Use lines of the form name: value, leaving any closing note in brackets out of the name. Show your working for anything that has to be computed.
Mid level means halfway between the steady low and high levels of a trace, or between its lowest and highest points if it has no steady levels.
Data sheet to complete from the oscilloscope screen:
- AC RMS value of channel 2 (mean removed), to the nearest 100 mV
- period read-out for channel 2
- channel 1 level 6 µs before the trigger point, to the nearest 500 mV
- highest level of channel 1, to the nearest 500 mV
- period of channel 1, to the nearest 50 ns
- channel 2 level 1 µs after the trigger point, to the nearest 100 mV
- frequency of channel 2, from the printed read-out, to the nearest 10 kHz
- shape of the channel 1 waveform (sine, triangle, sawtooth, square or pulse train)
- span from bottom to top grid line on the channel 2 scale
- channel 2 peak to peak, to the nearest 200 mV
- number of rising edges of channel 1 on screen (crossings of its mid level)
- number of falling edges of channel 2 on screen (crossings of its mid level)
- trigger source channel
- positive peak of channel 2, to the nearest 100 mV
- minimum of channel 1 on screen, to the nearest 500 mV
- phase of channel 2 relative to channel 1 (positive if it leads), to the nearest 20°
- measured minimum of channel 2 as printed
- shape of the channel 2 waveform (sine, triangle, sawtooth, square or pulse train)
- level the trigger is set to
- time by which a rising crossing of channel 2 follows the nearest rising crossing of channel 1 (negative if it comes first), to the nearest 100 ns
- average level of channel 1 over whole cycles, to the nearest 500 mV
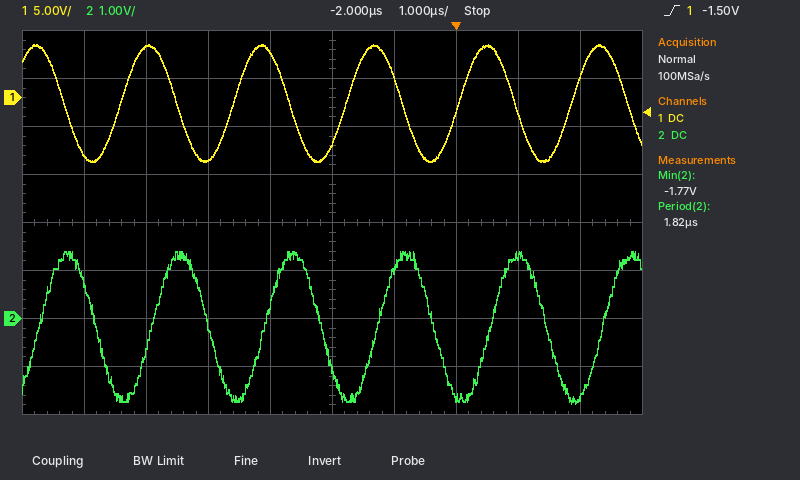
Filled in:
AC RMS value of channel 2 (mean removed), to the nearest 100 mV: 3.2 V / (2√2) ≈ 1.1 V
period read-out for channel 2: 1.82 µs
channel 1 level 6 µs before the trigger point, to the nearest 500 mV: -6.0 V
highest level of channel 1, to the nearest 500 mV: 5.5 V
period of channel 1, to the nearest 50 ns: 1.80 µs
channel 2 level 1 µs after the trigger point, to the nearest 100 mV: 1.3 V
frequency of channel 2, from the printed read-out, to the nearest 10 kHz: 1 / 1.82 µs ≈ 549 kHz, so 550 kHz to the nearest 10 kHz
shape of the channel 1 waveform: sine
span from bottom to top grid line on the channel 2 scale: 8 V
channel 2 peak to peak, to the nearest 200 mV: 3.2 V
number of rising edges of channel 1 on screen: 5
number of falling edges of channel 2 on screen: 5
trigger source channel: channel 1
positive peak of channel 2, to the nearest 100 mV: 1.4 V
minimum of channel 1 on screen, to the nearest 500 mV: -6.5 V
phase of channel 2 relative to channel 1 (positive if it leads), to the nearest 20°: −360° × (+500 ns) / 1.80 µs ≈ -100°
measured minimum of channel 2 as printed: -1.77 V
shape of the channel 2 waveform: sine
level the trigger is set to: -1.50 V
time by which a rising crossing of channel 2 follows the nearest rising crossing of channel 1 (negative if it comes first), to the nearest 100 ns: +500 ns
average level of channel 1 over whole cycles, to the nearest 500 mV: (5.5 V + (-6.5 V)) / 2 ≈ -500 mV
